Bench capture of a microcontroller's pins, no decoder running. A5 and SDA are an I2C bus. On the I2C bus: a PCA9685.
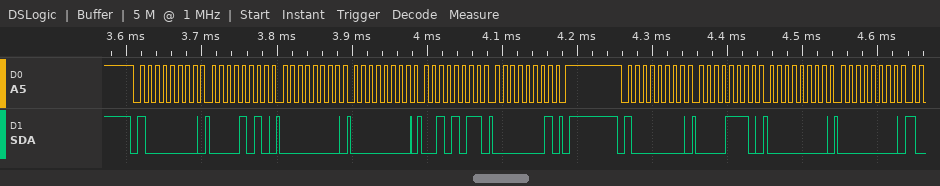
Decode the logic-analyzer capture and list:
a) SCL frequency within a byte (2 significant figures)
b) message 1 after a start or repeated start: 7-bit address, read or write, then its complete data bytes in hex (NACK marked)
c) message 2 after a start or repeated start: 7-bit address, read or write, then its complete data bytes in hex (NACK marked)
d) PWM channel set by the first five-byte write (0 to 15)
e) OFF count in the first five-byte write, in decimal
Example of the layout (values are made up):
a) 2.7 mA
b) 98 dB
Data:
a) 100 kHz
b) 0x40 write: 0A 00 00 2B 01
c) 0x40 write: 0E 00 00
d) 1
e) 299
